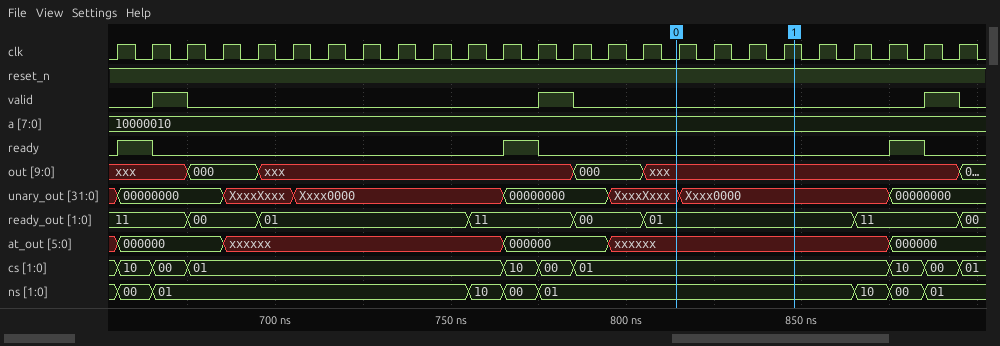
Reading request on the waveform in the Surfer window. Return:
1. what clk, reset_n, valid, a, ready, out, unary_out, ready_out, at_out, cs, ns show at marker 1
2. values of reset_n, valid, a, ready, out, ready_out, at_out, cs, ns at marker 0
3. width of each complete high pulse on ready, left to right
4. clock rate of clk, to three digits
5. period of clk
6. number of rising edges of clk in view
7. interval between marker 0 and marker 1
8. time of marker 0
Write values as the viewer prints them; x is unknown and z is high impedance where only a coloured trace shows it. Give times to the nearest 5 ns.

clk=1, reset_n=1, valid=0, a=10000010, ready=0, out=xxx, unary_out=Xxxx0000, ready_out=01, at_out=xxxxxx, cs=01, ns=01
reset_n=1, valid=0, a=10000010, ready=0, out=xxx, ready_out=01, at_out=xxxxxx, cs=01, ns=01
10 ns, 10 ns, 10 ns
100 MHz
10 ns
25
35 ns
815 ns
